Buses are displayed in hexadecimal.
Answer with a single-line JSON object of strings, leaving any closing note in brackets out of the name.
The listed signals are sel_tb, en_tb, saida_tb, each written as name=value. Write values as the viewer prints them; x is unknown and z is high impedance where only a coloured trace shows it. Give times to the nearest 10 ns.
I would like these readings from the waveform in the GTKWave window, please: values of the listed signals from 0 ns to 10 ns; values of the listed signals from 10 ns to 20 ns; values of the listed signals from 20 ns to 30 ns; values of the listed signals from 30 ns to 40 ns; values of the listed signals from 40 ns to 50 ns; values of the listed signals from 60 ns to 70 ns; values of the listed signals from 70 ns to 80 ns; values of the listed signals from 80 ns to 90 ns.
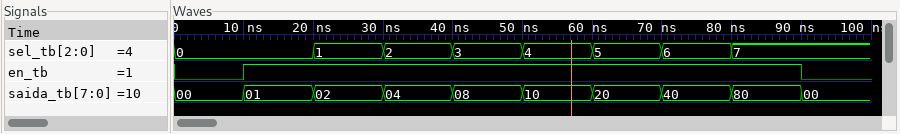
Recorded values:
{"values of the listed signals from 0 ns to 10 ns": "sel_tb=0, en_tb=0, saida_tb=00", "values of the listed signals from 10 ns to 20 ns": "sel_tb=0, en_tb=1, saida_tb=01", "values of the listed signals from 20 ns to 30 ns": "sel_tb=1, en_tb=1, saida_tb=02", "values of the listed signals from 30 ns to 40 ns": "sel_tb=2, en_tb=1, saida_tb=04", "values of the listed signals from 40 ns to 50 ns": "sel_tb=3, en_tb=1, saida_tb=08", "values of the listed signals from 60 ns to 70 ns": "sel_tb=5, en_tb=1, saida_tb=20", "values of the listed signals from 70 ns to 80 ns": "sel_tb=6, en_tb=1, saida_tb=40", "values of the listed signals from 80 ns to 90 ns": "sel_tb=7, en_tb=1, saida_tb=80"}
